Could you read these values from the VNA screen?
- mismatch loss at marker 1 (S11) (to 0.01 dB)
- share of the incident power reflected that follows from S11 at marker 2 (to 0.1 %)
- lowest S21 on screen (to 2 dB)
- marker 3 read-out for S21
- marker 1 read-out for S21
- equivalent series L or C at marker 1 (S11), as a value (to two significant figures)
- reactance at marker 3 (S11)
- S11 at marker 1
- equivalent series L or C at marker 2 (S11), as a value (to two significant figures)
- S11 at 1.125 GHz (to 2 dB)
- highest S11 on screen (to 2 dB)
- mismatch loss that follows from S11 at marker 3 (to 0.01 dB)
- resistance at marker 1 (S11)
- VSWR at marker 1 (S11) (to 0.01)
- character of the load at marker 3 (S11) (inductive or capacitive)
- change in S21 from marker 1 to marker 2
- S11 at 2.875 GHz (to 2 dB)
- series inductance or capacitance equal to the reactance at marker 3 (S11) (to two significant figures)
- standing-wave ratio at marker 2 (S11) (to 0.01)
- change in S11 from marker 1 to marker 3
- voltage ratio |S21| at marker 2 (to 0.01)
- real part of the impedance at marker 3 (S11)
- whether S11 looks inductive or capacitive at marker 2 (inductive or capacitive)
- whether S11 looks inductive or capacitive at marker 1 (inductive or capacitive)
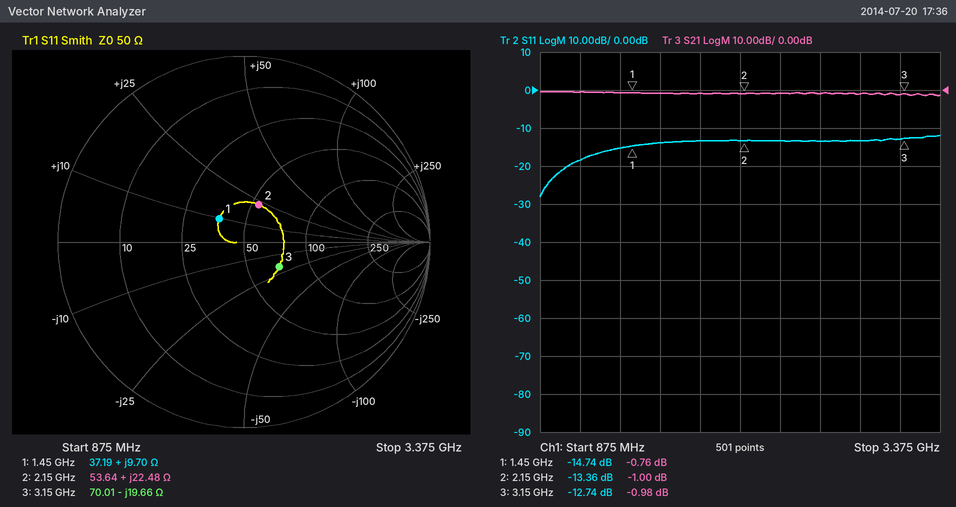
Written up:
0.15 dB
4.6 %
-2 dB
-0.98 dB
-0.76 dB
1.1 nH
-19.66 Ω
-14.74 dB
1.7 nH
-18 dB
-12 dB
0.24 dB
37.19 Ω
1.45
capacitive
-0.24 dB
-14 dB
2.6 pF
1.55
2.00 dB
0.89
70.01 Ω
inductive
inductive
